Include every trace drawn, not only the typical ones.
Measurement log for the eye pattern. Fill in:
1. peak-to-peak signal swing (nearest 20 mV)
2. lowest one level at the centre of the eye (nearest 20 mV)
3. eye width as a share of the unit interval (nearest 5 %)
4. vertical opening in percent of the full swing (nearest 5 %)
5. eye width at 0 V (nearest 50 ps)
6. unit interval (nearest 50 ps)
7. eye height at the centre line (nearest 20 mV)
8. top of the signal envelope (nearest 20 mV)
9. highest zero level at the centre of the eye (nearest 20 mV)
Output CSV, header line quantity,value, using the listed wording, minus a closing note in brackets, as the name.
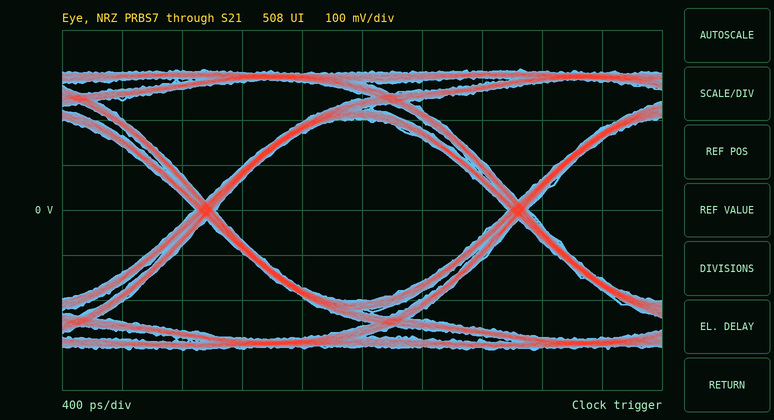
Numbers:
quantity,value
peak-to-peak signal swing,620 mV
lowest one level at the centre of the eye,200 mV
eye width as a share of the unit interval,95 %
vertical opening in percent of the full swing,65 %
eye width at 0 V,1.95 ns
unit interval,2.10 ns
eye height at the centre line,400 mV
top of the signal envelope,320 mV
highest zero level at the centre of the eye,-200 mV
